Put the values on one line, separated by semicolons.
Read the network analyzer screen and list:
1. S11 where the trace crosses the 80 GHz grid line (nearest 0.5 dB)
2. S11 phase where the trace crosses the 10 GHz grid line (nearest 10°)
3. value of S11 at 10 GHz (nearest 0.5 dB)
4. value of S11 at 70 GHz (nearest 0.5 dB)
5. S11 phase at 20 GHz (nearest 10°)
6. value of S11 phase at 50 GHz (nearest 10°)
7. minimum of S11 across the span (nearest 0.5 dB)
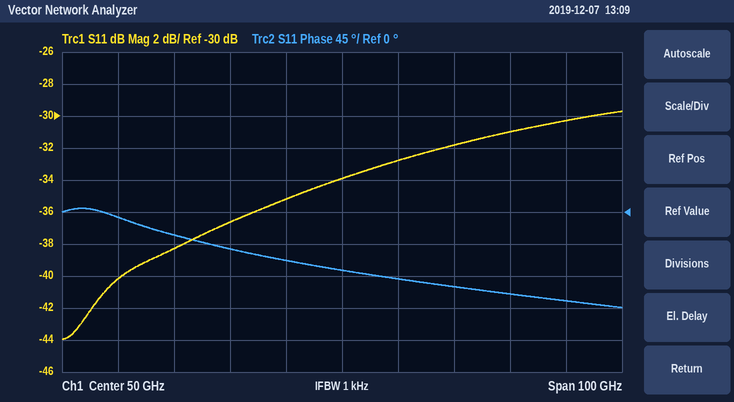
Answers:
-31.0 dB; -10°; -40.0 dB; -32.0 dB; -30°; -80°; -44.0 dB
